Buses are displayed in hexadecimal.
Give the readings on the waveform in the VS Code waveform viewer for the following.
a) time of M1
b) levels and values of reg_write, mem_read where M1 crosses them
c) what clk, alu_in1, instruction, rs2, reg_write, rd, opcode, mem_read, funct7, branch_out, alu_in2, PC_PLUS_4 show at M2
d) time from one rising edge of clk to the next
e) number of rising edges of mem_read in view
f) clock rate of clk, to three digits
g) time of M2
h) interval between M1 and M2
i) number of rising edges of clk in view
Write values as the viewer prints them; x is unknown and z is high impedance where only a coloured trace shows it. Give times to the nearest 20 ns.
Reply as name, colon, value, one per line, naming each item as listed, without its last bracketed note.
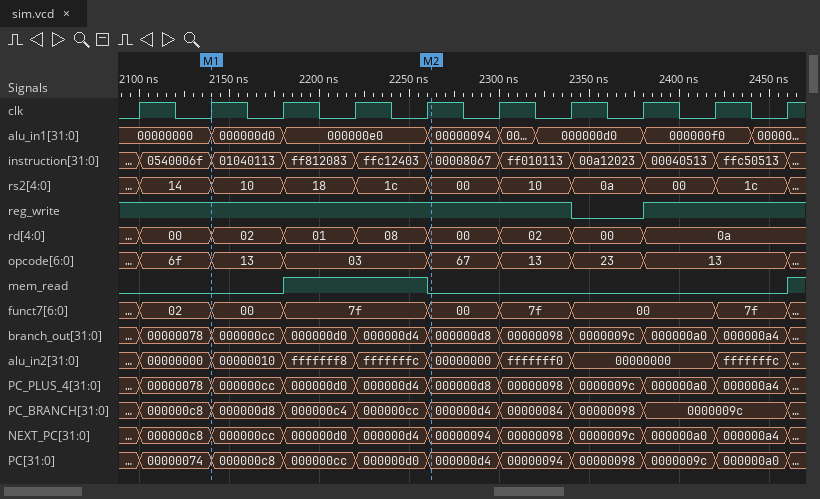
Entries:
time of M1: 2140 ns
levels and values of reg_write, mem_read where M1 crosses them: reg_write=1, mem_read=0
what clk, alu_in1, instruction, rs2, reg_write, rd, opcode, mem_read, funct7, branch_out, alu_in2, PC_PLUS_4 show at M2: clk=1, alu_in1=00000094, instruction=00008067, rs2=00, reg_write=1, rd=00, opcode=67, mem_read=0, funct7=00, branch_out=000000d8, alu_in2=00000000, PC_PLUS_4=000000d8
time from one rising edge of clk to the next: 40 ns
number of rising edges of mem_read in view: 2
clock rate of clk, to three digits: 25.0 MHz
time of M2: 2260 ns
interval between M1 and M2: 120 ns
number of rising edges of clk in view: 10
